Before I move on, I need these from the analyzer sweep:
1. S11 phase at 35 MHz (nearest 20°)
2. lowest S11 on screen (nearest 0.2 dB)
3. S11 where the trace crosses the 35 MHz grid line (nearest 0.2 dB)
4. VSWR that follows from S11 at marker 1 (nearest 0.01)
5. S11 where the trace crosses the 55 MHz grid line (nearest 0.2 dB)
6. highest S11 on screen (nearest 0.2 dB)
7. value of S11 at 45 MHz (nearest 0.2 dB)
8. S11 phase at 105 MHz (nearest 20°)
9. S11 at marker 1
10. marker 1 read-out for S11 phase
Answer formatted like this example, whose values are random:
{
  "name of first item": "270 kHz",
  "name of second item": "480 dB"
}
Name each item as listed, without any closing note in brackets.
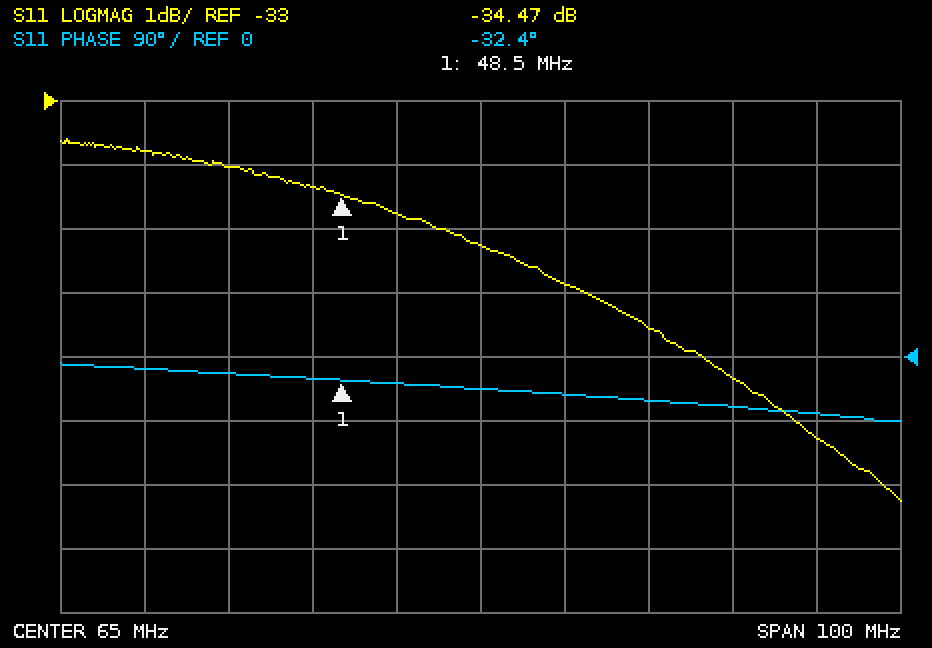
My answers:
{
  "S11 phase at 35 MHz": "-20°",
  "lowest S11 on screen": "-39.2 dB",
  "S11 where the trace crosses the 35 MHz grid line": "-34.0 dB",
  "VSWR that follows from S11 at marker 1": "1.04",
  "S11 where the trace crosses the 55 MHz grid line": "-34.8 dB",
  "highest S11 on screen": "-33.6 dB",
  "value of S11 at 45 MHz": "-34.4 dB",
  "S11 phase at 105 MHz": "-80°",
  "S11 at marker 1": "-34.47 dB",
  "marker 1 read-out for S11 phase": "-32.4°"
}
